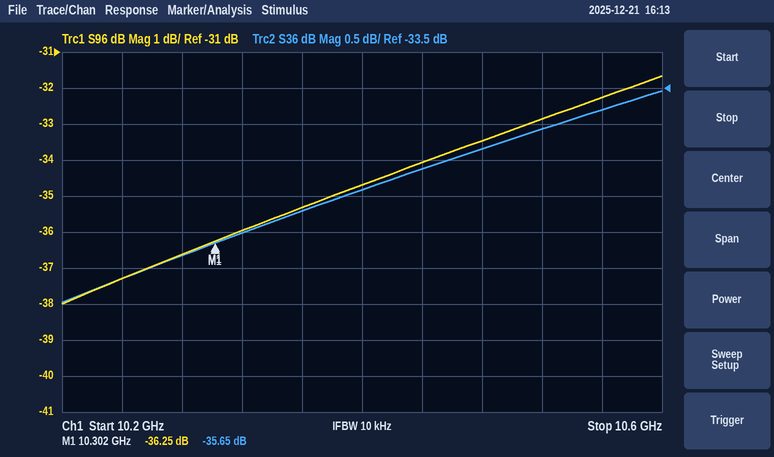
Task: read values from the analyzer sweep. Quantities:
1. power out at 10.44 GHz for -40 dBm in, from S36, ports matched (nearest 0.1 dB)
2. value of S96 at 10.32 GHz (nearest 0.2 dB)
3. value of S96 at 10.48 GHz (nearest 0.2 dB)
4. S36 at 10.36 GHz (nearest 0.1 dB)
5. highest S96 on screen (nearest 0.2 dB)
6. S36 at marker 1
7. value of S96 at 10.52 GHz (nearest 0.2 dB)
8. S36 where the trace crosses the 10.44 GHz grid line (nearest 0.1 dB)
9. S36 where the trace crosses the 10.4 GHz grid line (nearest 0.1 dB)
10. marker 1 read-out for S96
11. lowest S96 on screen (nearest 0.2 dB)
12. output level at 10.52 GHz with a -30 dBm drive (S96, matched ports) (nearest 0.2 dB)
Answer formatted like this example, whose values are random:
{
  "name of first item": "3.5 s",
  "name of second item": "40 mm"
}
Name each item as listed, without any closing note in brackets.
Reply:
{
  "power out at 10.44 GHz for -40 dBm in, from S36, ports matched": "-74.6 dBm",
  "value of S96 at 10.32 GHz": "-36.0 dB",
  "value of S96 at 10.48 GHz": "-33.4 dB",
  "S36 at 10.36 GHz": "-35.2 dB",
  "highest S96 on screen": "-31.6 dB",
  "S36 at marker 1": "-35.65 dB",
  "value of S96 at 10.52 GHz": "-32.8 dB",
  "S36 where the trace crosses the 10.44 GHz grid line": "-34.6 dB",
  "S36 where the trace crosses the 10.4 GHz grid line": "-34.9 dB",
  "marker 1 read-out for S96": "-36.25 dB",
  "lowest S96 on screen": "-38.0 dB",
  "output level at 10.52 GHz with a -30 dBm drive (S96, matched ports)": "-62.8 dBm"
}
